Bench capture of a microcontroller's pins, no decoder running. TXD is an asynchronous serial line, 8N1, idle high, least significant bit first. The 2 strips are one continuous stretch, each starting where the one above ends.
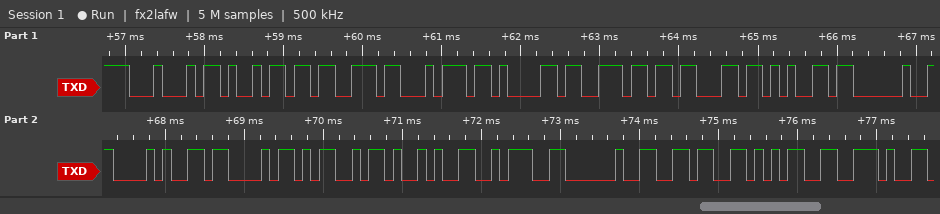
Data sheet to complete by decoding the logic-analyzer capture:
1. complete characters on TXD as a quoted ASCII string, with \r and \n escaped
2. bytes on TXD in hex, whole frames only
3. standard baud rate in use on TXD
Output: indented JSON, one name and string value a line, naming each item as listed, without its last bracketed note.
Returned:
{
  "complete characters on TXD as a quoted ASCII string, with \\r and \\n escaped": "\"Distance (CM): 65.\"",
  "bytes on TXD in hex, whole frames only": "44 69 73 74 61 6E 63 65 20 28 43 4D 29 3A 20 36 35 2E",
  "standard baud rate in use on TXD": "9600 baud"
}
